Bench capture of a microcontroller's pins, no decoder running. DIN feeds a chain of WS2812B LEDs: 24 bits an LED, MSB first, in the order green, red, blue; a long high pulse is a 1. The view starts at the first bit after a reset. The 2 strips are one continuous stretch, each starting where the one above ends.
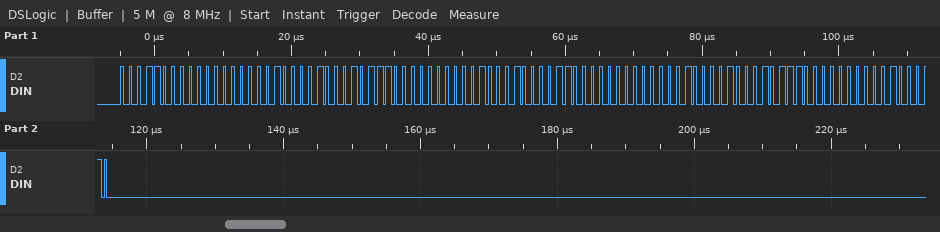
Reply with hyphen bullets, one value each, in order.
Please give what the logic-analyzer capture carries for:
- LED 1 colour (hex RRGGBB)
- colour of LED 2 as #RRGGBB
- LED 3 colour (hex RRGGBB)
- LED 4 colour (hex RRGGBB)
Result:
- #001821
- #001722
- #001821
- #001722
